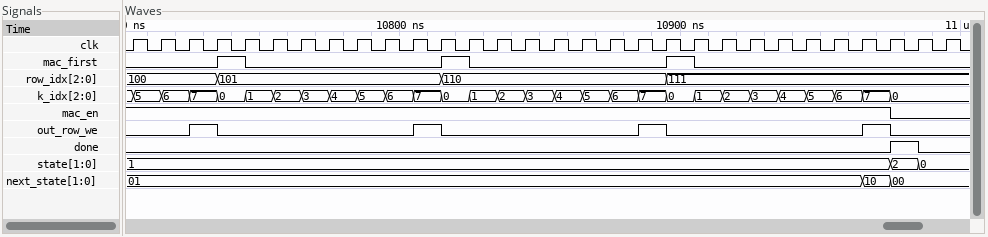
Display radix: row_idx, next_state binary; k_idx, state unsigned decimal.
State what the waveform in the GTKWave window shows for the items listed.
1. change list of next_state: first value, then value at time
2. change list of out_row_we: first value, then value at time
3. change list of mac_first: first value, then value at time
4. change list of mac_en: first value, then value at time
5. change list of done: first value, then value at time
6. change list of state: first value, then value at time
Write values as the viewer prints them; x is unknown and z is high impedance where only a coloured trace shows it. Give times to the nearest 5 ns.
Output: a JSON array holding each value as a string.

["01, 10 at 10965 ns, 00 at 10975 ns", "0, 1 at 10725 ns, 0 at 10735 ns, 1 at 10805 ns, 0 at 10815 ns, 1 at 10885 ns, 0 at 10895 ns, 1 at 10965 ns, 0 at 10975 ns", "0, 1 at 10735 ns, 0 at 10745 ns, 1 at 10815 ns, 0 at 10825 ns, 1 at 10895 ns, 0 at 10905 ns", "1, 0 at 10975 ns", "0, 1 at 10975 ns, 0 at 10985 ns", "1, 2 at 10975 ns, 0 at 10985 ns"]
